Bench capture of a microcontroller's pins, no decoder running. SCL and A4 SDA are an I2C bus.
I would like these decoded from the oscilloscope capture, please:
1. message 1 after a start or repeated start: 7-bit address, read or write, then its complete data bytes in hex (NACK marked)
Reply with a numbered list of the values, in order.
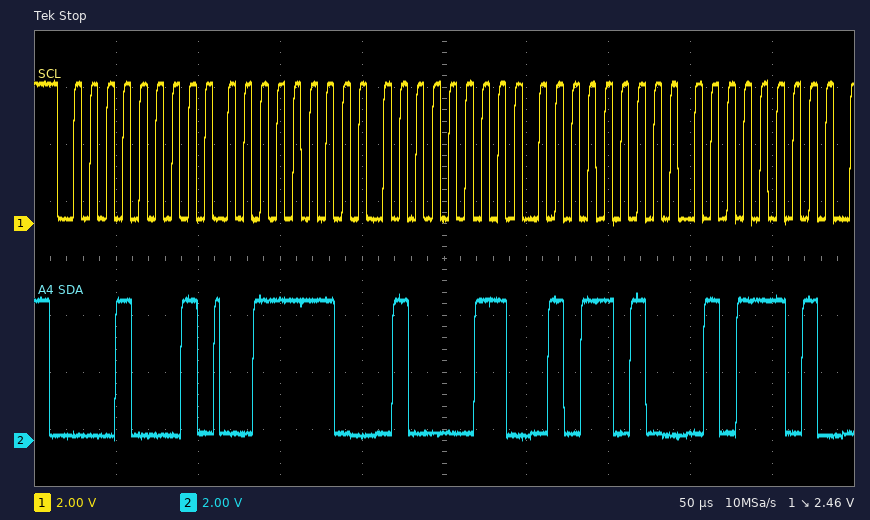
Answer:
1. 0x08 read: 3E 43 5A 5D
